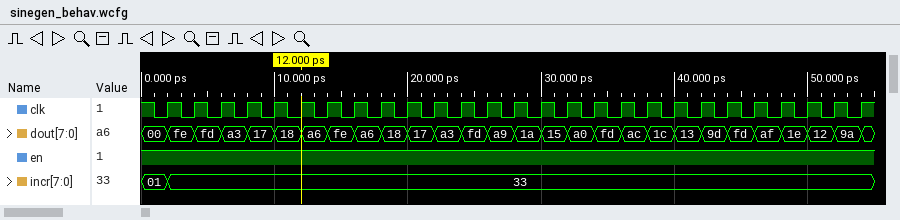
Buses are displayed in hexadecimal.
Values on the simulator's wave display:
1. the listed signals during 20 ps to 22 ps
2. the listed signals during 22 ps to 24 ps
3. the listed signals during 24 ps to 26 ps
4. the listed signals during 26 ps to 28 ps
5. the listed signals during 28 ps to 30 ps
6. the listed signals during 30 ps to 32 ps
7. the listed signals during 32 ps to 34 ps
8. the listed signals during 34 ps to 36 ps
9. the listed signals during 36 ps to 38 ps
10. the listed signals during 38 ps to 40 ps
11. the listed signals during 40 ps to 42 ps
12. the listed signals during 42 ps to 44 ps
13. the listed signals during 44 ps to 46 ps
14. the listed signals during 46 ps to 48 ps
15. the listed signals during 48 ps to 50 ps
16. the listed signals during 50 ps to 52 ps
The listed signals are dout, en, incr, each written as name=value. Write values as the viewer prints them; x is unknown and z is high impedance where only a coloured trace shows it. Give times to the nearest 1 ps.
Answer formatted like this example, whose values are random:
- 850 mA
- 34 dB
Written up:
- dout=17, en=1, incr=33
- dout=a3, en=1, incr=33
- dout=fd, en=1, incr=33
- dout=a9, en=1, incr=33
- dout=1a, en=1, incr=33
- dout=15, en=1, incr=33
- dout=a0, en=1, incr=33
- dout=fd, en=1, incr=33
- dout=ac, en=1, incr=33
- dout=1c, en=1, incr=33
- dout=13, en=1, incr=33
- dout=9d, en=1, incr=33
- dout=fd, en=1, incr=33
- dout=af, en=1, incr=33
- dout=1e, en=1, incr=33
- dout=12, en=1, incr=33
